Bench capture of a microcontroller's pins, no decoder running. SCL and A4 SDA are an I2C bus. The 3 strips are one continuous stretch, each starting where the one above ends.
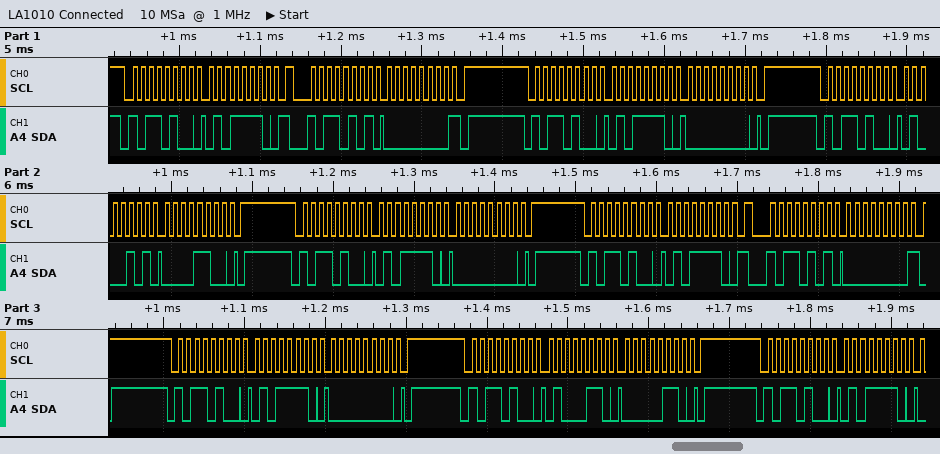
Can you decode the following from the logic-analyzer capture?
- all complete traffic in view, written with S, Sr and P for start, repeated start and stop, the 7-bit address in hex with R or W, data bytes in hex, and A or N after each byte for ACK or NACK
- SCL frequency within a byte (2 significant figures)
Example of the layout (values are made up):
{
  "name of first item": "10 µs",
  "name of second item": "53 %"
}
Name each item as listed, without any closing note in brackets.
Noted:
{
  "all complete traffic in view, written with S, Sr and P for start, repeated start and stop, the 7-bit address in hex with R or W, data bytes in hex, and A or N after each byte for ACK or NACK": "S 5AW A 5E A Sr 5AR A 00 N P S 5AW A 5E A 00 A P S 5AW A 45 A 0C A P S 5AW A 5E A 00 A P S 5AW A 5E A Sr 5AR A 00 N P S 5AW A 5E A 00 A P S 5AW A 46 A 06 A P S 5AW A 5E A",
  "SCL frequency within a byte": "100 kHz"
}
